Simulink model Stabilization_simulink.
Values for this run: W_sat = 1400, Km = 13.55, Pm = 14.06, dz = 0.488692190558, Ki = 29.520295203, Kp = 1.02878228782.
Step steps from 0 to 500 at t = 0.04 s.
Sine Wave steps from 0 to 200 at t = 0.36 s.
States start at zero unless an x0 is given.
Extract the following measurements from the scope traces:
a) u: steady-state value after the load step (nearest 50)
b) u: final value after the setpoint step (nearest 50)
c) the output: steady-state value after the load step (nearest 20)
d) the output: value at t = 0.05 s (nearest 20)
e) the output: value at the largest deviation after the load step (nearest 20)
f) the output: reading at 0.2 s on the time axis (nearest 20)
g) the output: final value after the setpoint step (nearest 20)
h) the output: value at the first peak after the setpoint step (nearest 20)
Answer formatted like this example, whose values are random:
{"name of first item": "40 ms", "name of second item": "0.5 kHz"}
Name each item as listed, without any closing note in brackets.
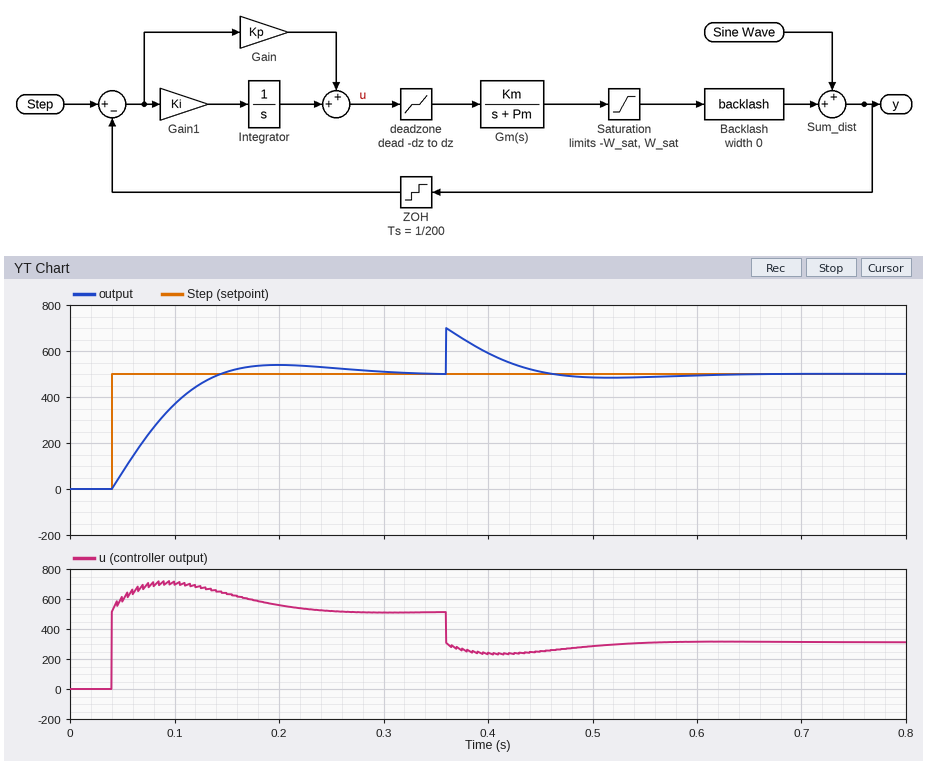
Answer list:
{"u: steady-state value after the load step": "300", "u: final value after the setpoint step": "500", "the output: steady-state value after the load step": "500", "the output: value at t = 0.05 s": "80", "the output: value at the largest deviation after the load step": "700", "the output: reading at 0.2 s on the time axis": "540", "the output: final value after the setpoint step": "500", "the output: value at the first peak after the setpoint step": "540"}
